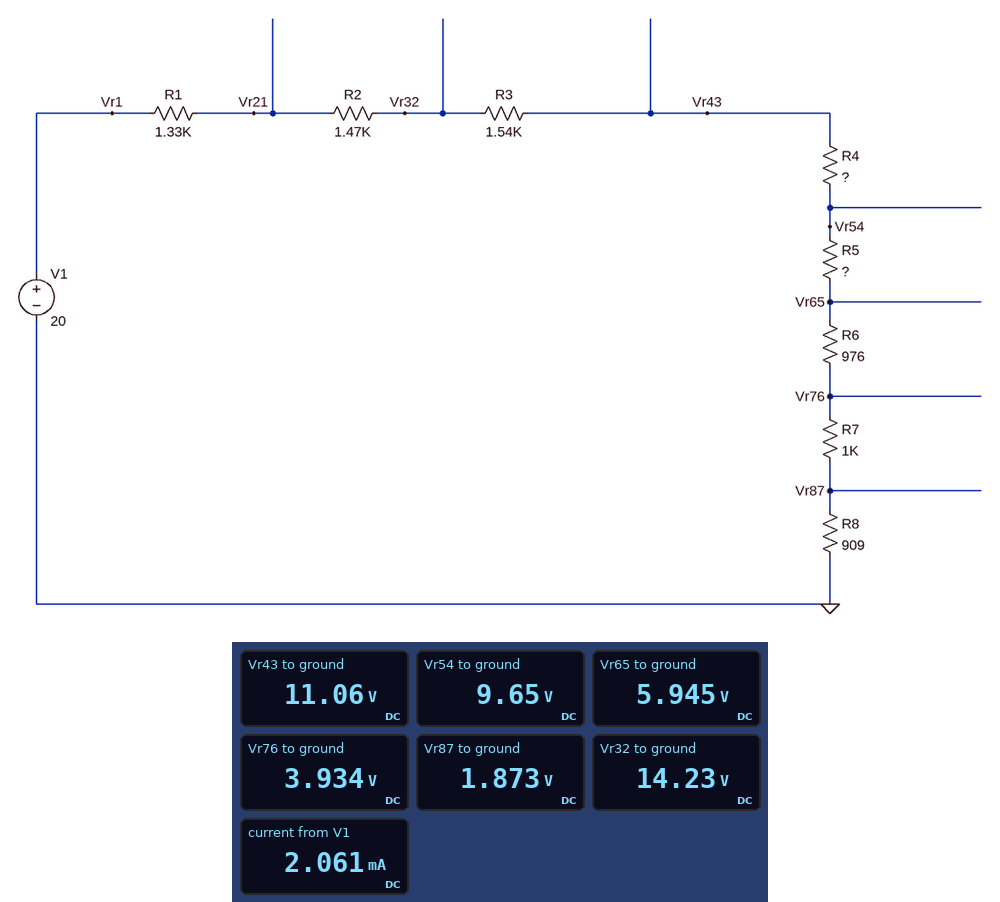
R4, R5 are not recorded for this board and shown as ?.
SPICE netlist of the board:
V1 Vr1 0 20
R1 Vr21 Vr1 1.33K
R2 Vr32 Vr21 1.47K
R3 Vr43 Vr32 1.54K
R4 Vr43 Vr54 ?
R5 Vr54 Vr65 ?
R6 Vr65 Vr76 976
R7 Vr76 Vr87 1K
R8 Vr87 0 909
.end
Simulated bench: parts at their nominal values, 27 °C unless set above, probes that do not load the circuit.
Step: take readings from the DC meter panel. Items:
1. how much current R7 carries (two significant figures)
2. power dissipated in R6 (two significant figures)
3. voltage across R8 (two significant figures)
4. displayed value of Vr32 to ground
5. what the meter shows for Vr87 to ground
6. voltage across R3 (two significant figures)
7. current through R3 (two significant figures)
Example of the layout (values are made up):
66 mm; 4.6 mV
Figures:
2.1 mA; 4.1 mW; 1.9 V; 14.23 V; 1.873 V; 3.2 V; 2.1 mA
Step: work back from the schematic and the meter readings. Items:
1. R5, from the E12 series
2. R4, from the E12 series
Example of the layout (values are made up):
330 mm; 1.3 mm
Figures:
1.8 kΩ; 680 Ω
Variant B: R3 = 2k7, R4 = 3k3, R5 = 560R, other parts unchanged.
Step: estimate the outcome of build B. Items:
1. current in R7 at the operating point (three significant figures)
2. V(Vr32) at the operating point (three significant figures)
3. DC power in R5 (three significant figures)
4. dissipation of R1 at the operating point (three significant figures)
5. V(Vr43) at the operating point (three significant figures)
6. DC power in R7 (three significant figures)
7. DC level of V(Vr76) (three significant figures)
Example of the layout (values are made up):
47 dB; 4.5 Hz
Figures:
1.63 mA; 15.4 V; 1.49 mW; 3.55 mW; 11.0 V; 2.67 mW; 3.12 V
